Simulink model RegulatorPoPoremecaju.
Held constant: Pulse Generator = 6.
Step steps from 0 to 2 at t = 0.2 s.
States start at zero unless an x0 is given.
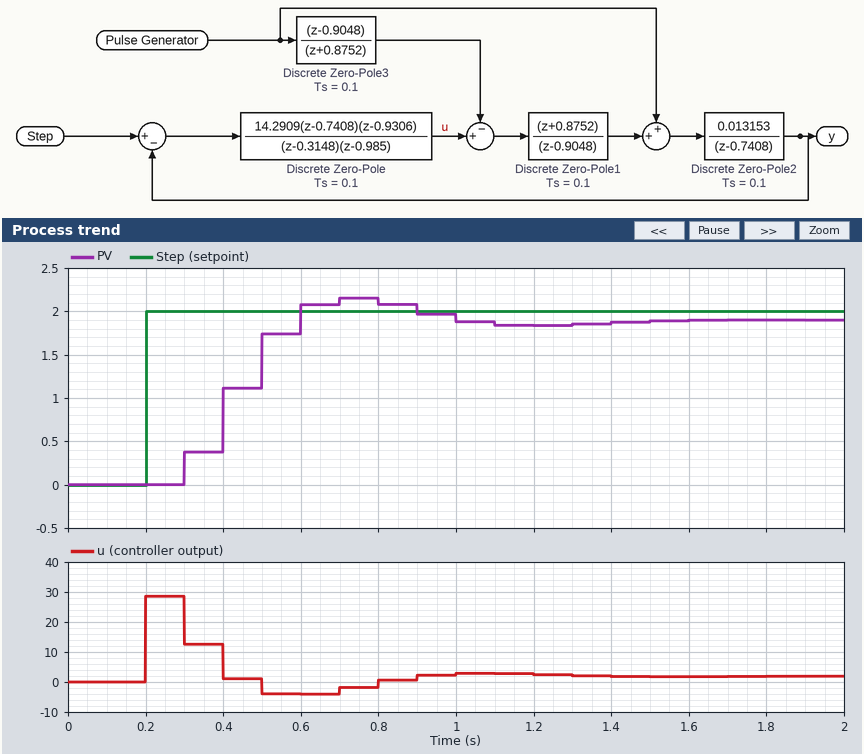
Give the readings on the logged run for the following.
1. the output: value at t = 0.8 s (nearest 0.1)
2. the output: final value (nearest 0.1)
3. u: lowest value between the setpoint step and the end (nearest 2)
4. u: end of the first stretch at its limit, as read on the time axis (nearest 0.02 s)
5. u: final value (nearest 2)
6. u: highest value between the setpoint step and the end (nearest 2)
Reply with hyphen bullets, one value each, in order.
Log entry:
- 2.1
- 1.9
- -4
- 0.30 s
- 2
- 28
